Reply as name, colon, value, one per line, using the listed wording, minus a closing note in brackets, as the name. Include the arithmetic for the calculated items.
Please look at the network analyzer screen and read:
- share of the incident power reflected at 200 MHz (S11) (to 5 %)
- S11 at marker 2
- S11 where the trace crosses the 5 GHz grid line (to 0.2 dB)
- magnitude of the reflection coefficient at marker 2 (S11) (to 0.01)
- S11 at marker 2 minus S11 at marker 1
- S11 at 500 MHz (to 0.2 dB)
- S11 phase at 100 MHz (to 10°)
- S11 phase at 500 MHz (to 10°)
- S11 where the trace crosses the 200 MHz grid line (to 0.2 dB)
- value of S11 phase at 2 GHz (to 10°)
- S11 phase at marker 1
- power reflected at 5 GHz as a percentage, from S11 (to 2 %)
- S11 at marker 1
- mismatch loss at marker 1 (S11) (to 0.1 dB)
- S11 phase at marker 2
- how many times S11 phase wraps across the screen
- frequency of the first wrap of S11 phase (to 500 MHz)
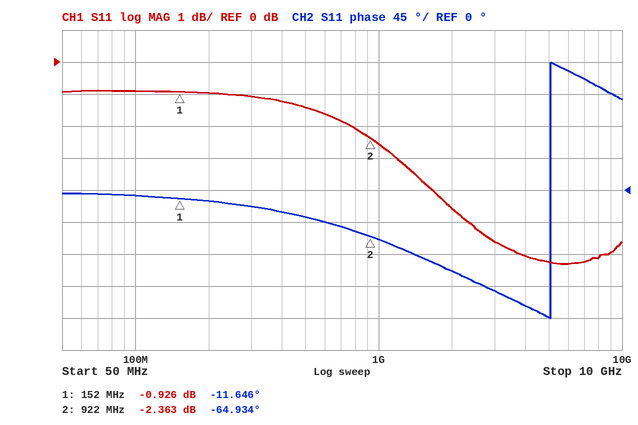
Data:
share of the incident power reflected at 200 MHz (S11): 10^(-1/10) ≈ 79.4 %, so 80 % to the nearest 5 %
S11 at marker 2: -2.363 dB
S11 where the trace crosses the 5 GHz grid line: -6.2 dB
magnitude of the reflection coefficient at marker 2 (S11): 10^(-2.363/20) ≈ 0.76
S11 at marker 2 minus S11 at marker 1: -2.363 − (-0.926) = -1.437 dB
S11 at 500 MHz: -1.4 dB
S11 phase at 100 MHz: -10°
S11 phase at 500 MHz: -40°
S11 where the trace crosses the 200 MHz grid line: -1.0 dB
value of S11 phase at 2 GHz: -110°
S11 phase at marker 1: -11.646°
power reflected at 5 GHz as a percentage, from S11: 10^(-6.2/10) ≈ 24 %
S11 at marker 1: -0.926 dB
mismatch loss at marker 1 (S11): −10 log10(1 − 10^(-0.926/10)) ≈ 7.2 dB
S11 phase at marker 2: -64.934°
how many times S11 phase wraps across the screen: 1
frequency of the first wrap of S11 phase: 5.0 GHz
